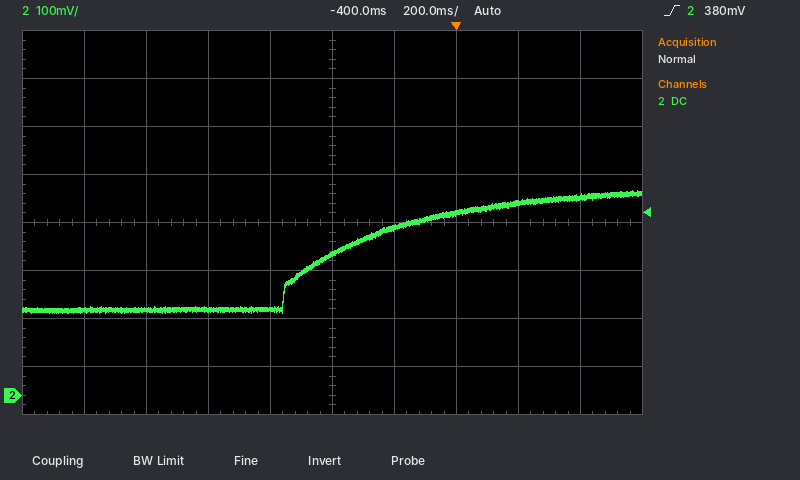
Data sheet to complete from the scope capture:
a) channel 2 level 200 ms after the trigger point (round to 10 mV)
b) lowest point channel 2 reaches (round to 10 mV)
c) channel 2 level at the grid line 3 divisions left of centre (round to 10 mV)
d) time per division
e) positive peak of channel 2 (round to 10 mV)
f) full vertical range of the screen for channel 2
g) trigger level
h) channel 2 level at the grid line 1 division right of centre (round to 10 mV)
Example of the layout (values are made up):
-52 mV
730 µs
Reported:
400 mV
170 mV
180 mV
200 ms
430 mV
800 mV
380 mV
350 mV
